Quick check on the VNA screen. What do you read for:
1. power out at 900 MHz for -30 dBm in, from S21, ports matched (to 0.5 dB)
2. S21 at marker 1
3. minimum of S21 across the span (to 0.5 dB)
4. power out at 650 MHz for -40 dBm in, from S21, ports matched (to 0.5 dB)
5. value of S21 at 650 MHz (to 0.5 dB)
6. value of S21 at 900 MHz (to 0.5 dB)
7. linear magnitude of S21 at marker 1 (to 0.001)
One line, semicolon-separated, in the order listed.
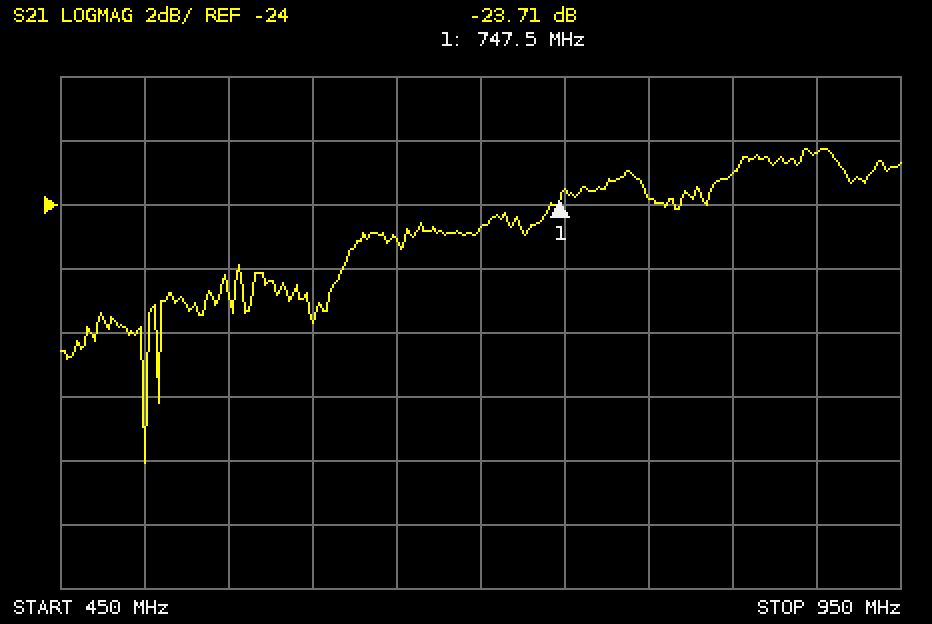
-52.5 dBm; -23.71 dB; -32.0 dB; -65.0 dBm; -25.0 dB; -22.5 dB; 0.065
